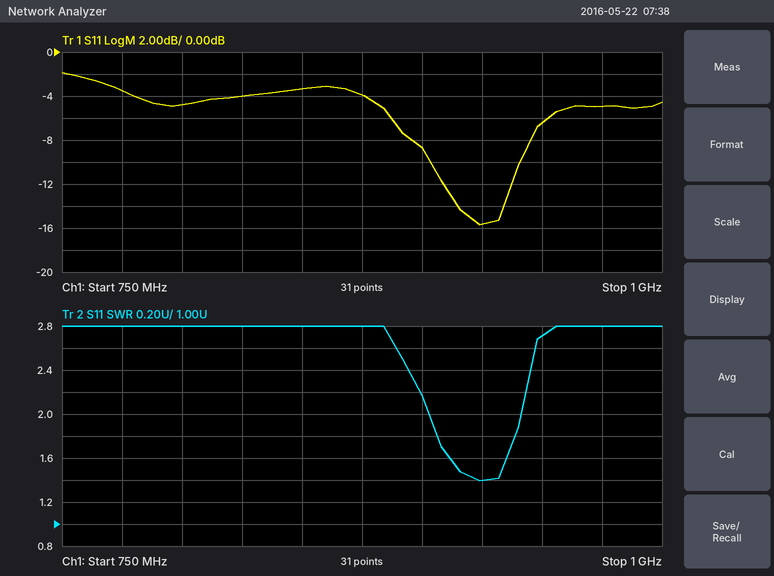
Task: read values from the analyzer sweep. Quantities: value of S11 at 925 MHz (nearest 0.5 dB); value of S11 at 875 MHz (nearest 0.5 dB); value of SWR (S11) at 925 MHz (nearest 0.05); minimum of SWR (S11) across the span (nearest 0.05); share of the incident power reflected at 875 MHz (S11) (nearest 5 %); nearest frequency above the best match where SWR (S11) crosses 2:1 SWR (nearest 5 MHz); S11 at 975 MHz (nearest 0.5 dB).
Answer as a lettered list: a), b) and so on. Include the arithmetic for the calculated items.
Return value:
a) -15.5 dB
b) -4.0 dB
c) 1.40
d) 1.40
e) 10^(-4/10) ≈ 40 %
f) 940 MHz
g) -5.0 dB
